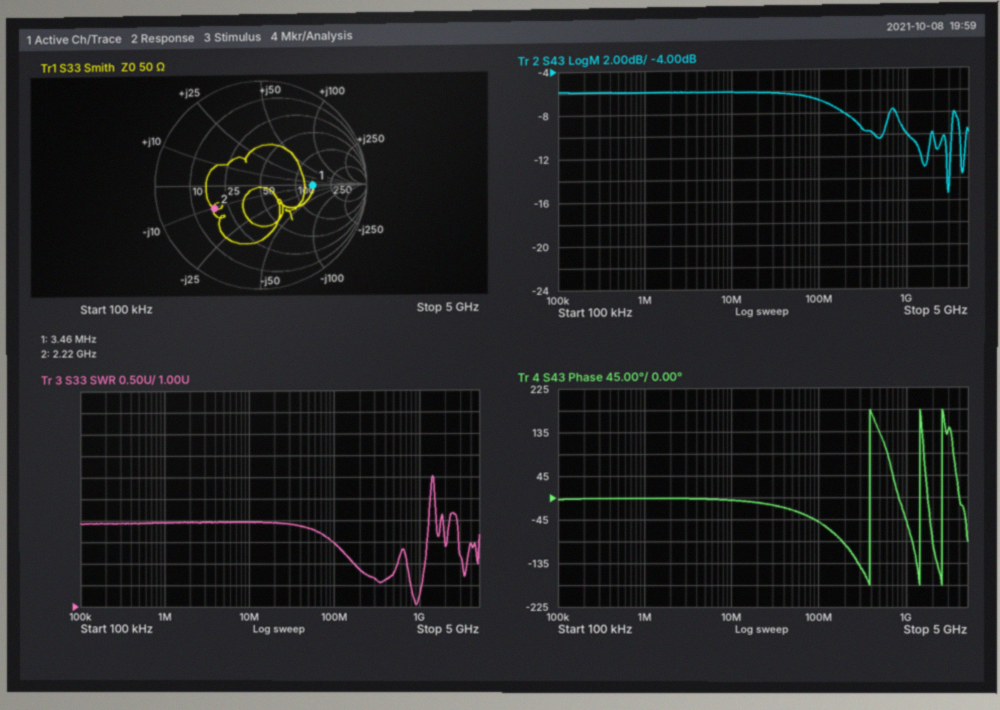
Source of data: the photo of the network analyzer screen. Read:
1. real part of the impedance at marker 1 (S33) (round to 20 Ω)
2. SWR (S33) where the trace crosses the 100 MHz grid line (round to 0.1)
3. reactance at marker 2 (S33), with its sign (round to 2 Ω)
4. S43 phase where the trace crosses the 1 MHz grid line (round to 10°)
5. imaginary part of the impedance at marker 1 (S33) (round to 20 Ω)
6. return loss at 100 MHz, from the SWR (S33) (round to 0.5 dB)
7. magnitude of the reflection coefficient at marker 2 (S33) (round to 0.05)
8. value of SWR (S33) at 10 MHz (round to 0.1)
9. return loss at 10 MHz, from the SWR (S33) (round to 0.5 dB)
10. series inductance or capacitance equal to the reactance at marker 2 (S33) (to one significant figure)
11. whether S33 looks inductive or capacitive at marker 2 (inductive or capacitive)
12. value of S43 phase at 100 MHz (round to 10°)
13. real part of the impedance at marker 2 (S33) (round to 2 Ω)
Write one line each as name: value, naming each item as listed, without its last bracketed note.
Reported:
real part of the impedance at marker 1 (S33): 140 Ω
SWR (S33) where the trace crosses the 100 MHz grid line: 2.5
reactance at marker 2 (S33), with its sign: -10 Ω
S43 phase where the trace crosses the 1 MHz grid line: 0°
imaginary part of the impedance at marker 1 (S33): 0 Ω
return loss at 100 MHz, from the SWR (S33): 7.5 dB
magnitude of the reflection coefficient at marker 2 (S33): 0.50
value of SWR (S33) at 10 MHz: 3.0
return loss at 10 MHz, from the SWR (S33): 6.0 dB
series inductance or capacitance equal to the reactance at marker 2 (S33): 7 pF
whether S33 looks inductive or capacitive at marker 2: capacitive
value of S43 phase at 100 MHz: -50°
real part of the impedance at marker 2 (S33): 18 Ω
